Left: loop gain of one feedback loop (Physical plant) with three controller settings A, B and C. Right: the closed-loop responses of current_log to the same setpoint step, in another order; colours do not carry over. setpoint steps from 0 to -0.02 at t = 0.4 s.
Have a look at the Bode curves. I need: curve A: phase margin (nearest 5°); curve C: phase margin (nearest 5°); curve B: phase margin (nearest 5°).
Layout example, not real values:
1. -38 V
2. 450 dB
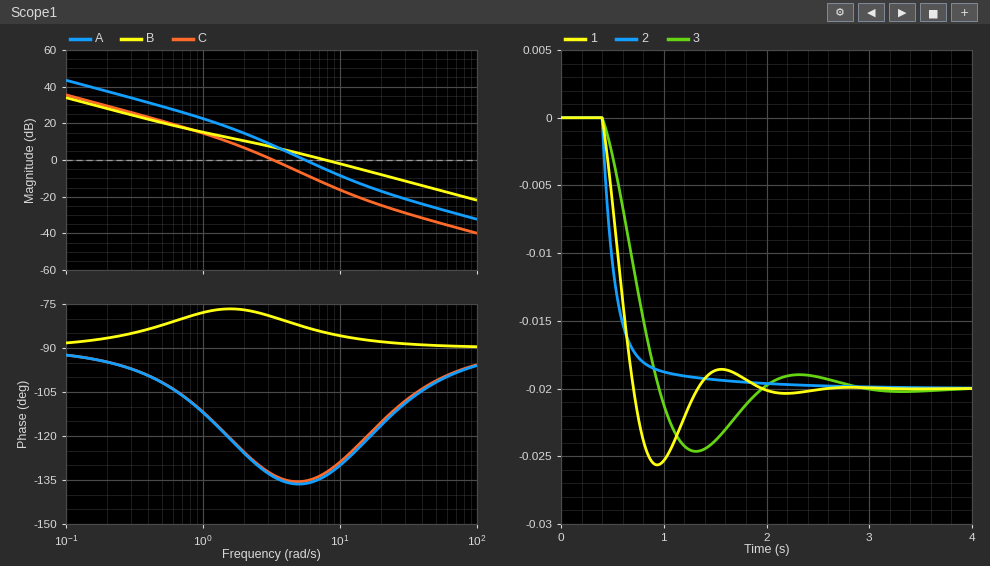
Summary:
1. 45°
2. 45°
3. 95°
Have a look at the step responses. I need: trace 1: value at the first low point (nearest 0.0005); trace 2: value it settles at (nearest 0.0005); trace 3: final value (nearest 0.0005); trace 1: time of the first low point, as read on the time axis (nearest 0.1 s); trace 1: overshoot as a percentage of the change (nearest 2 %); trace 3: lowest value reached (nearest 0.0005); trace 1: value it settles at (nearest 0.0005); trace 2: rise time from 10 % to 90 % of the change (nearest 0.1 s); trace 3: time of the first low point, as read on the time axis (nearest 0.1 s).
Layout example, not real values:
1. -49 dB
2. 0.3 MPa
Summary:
1. -0.0255
2. -0.0200
3. -0.0200
4. 0.9 s
5. 28 %
6. -0.0245
7. -0.0200
8. 0.4 s
9. 1.3 s
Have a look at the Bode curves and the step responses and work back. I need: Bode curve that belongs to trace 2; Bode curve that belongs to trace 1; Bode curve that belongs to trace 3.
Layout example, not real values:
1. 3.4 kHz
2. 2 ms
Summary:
1. B
2. A
3. C
